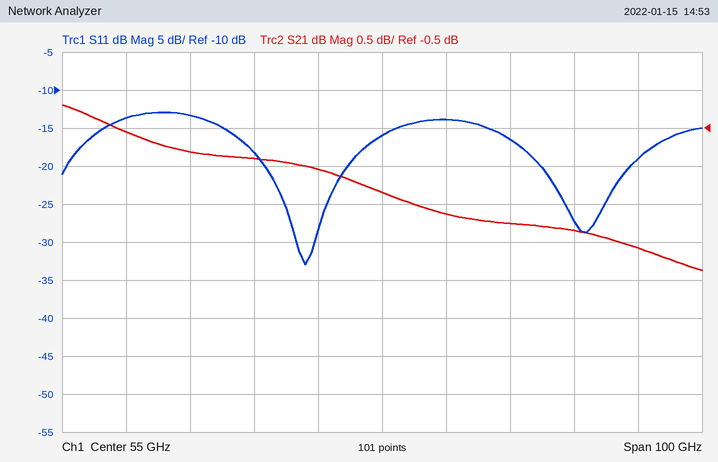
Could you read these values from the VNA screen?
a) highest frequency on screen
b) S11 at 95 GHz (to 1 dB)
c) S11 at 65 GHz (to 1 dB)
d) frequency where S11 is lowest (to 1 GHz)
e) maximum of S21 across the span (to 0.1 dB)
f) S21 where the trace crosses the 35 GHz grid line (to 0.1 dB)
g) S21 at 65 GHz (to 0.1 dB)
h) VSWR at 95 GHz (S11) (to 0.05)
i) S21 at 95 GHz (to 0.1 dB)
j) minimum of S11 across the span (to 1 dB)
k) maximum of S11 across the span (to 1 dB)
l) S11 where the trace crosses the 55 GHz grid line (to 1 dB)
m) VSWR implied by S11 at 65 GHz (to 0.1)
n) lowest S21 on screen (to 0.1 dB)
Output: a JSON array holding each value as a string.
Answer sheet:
["105 GHz", "-19 dB", "-14 dB", "43 GHz", "-0.2 dB", "-0.9 dB", "-1.6 dB", "1.25", "-2.1 dB", "-33 dB", "-13 dB", "-16 dB", "1.5", "-2.4 dB"]
